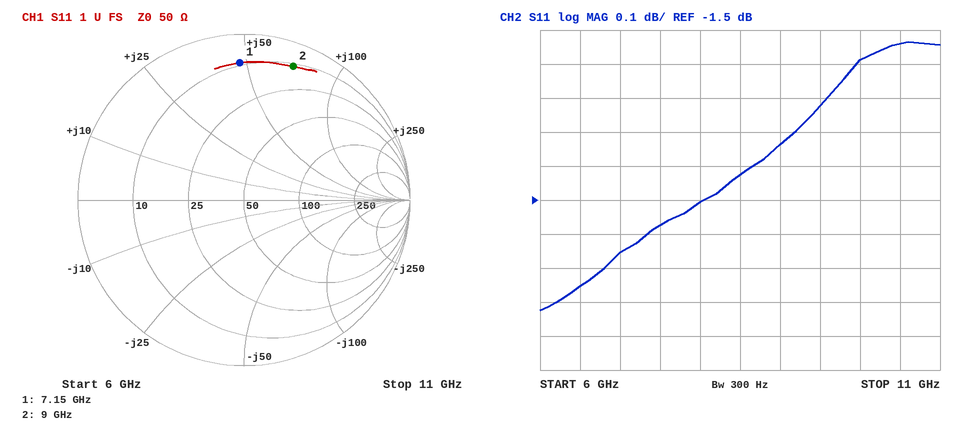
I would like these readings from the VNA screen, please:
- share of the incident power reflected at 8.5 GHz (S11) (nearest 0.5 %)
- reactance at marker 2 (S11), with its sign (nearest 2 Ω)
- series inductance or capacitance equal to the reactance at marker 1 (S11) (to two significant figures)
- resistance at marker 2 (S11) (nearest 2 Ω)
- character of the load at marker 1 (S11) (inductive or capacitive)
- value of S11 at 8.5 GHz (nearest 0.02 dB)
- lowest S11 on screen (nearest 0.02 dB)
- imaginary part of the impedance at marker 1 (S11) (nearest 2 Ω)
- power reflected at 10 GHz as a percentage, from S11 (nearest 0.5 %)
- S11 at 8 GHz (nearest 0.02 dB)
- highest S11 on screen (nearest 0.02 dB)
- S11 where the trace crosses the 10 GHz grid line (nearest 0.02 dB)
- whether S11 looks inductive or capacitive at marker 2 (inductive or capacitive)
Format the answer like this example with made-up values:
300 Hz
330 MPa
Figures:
72.0 %
+70 Ω
1.1 nH
12 Ω
inductive
-1.42 dB
-1.82 dB
+48 Ω
78.0 %
-1.50 dB
-1.04 dB
-1.08 dB
inductive
